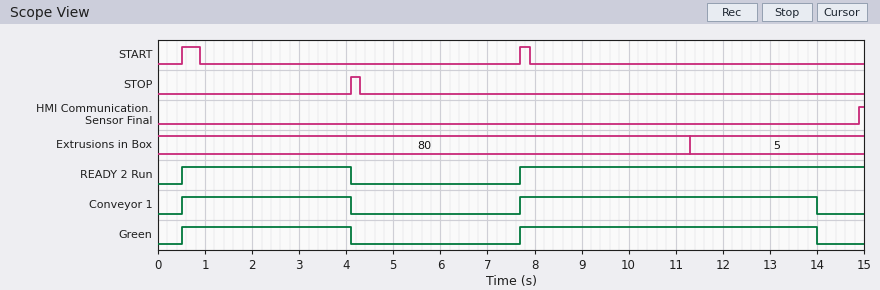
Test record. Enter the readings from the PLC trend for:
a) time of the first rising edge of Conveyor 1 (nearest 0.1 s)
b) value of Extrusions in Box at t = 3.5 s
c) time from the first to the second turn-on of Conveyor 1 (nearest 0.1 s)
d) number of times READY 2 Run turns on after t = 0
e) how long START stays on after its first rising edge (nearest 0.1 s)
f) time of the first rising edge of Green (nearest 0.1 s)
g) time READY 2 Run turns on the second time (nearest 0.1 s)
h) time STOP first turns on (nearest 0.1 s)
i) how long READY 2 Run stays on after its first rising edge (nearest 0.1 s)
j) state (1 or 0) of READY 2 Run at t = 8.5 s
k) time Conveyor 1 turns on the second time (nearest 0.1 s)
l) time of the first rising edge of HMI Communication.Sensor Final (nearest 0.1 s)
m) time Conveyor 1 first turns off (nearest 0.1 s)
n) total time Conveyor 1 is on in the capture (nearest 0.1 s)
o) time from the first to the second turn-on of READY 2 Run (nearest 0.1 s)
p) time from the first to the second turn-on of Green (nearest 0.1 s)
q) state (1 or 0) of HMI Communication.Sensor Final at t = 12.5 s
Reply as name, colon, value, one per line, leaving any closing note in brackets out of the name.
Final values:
time of the first rising edge of Conveyor 1: 0.5 s
value of Extrusions in Box at t = 3.5 s: 80
time from the first to the second turn-on of Conveyor 1: 7.2 s
number of times READY 2 Run turns on after t = 0: 2
how long START stays on after its first rising edge: 0.4 s
time of the first rising edge of Green: 0.5 s
time READY 2 Run turns on the second time: 7.7 s
time STOP first turns on: 4.1 s
how long READY 2 Run stays on after its first rising edge: 3.6 s
state (1 or 0) of READY 2 Run at t = 8.5 s: 1
time Conveyor 1 turns on the second time: 7.7 s
time of the first rising edge of HMI Communication.Sensor Final: 14.9 s
time Conveyor 1 first turns off: 4.1 s
total time Conveyor 1 is on in the capture: 9.9 s
time from the first to the second turn-on of READY 2 Run: 7.2 s
time from the first to the second turn-on of Green: 7.2 s
state (1 or 0) of HMI Communication.Sensor Final at t = 12.5 s: 0
